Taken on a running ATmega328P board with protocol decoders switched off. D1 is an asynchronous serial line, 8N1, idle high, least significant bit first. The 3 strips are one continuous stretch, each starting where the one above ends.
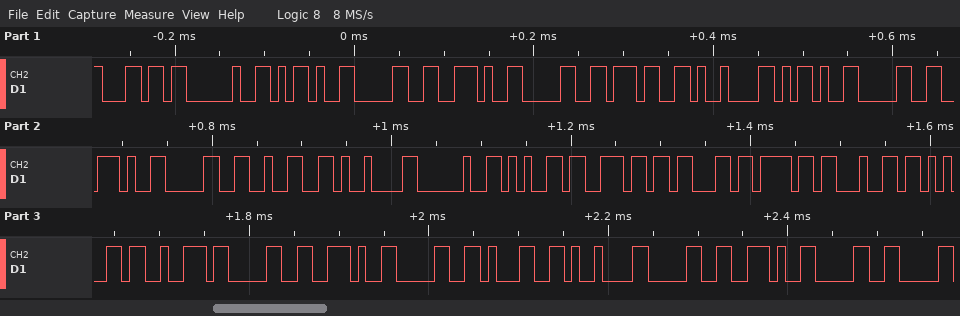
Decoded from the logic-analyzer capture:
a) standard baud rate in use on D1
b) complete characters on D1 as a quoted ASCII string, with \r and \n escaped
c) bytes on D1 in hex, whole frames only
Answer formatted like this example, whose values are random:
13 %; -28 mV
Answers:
115200 baud; "l -0.07\t-0.02\t encoder0.01\t0.0"; 0x6C 0x20 0x2D 0x30 0x2E 0x30 0x37 0x09 0x2D 0x30 0x2E 0x30 0x32 0x09 0x20 0x65 0x6E 0x63 0x6F 0x64 0x65 0x72 0x30 0x2E 0x30 0x31 0x09 0x30 0x2E 0x30
